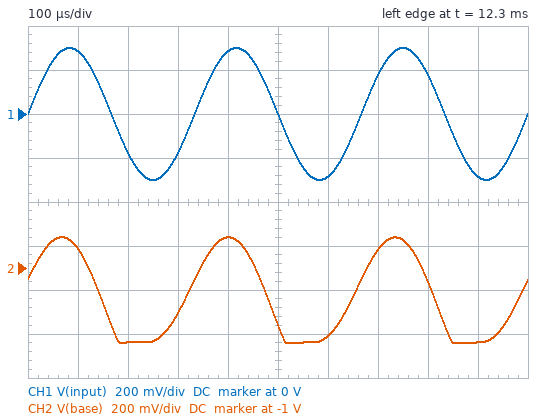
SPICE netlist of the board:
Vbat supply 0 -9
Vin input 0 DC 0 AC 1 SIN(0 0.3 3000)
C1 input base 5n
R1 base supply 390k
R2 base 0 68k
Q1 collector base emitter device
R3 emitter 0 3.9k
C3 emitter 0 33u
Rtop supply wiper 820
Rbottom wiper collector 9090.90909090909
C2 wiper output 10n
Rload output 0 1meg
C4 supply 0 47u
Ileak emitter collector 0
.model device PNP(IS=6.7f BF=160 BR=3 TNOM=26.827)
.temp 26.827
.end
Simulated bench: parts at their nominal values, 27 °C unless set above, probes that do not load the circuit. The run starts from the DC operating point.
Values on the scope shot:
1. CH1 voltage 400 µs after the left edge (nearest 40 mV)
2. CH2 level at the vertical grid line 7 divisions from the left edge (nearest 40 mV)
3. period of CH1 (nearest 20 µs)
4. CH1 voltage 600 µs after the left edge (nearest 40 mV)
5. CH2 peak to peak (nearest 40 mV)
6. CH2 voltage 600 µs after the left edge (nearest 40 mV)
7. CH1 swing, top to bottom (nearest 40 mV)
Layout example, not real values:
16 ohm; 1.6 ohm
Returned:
280 mV; -920 mV; 340 µs; -280 mV; 480 mV; -1.32 V; 600 mV
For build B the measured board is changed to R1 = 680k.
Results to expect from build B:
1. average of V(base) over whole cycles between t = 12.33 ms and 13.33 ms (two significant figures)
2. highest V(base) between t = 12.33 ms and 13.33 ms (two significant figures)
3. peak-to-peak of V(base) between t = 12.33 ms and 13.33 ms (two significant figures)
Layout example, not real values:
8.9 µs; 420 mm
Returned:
-680 mV; -400 mV; 530 mV
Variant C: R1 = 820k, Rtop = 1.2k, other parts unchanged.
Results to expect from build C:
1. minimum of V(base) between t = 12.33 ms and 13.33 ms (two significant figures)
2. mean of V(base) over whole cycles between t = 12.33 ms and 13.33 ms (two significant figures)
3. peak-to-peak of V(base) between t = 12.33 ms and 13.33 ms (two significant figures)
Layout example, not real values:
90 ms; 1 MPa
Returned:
-830 mV; -570 mV; 540 mV
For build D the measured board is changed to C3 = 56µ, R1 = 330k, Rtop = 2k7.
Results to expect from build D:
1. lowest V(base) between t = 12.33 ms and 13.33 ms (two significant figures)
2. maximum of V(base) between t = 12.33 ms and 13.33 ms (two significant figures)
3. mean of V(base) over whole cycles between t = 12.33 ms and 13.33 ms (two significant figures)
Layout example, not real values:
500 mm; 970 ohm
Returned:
-1.5 V; -1.0 V; -1.3 V
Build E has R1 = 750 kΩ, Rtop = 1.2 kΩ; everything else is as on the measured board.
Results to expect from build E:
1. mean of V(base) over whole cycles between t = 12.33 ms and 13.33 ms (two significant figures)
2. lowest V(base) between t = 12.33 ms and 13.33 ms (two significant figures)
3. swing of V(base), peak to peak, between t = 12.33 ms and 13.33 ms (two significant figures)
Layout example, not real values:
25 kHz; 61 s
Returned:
-620 mV; -870 mV; 530 mV
